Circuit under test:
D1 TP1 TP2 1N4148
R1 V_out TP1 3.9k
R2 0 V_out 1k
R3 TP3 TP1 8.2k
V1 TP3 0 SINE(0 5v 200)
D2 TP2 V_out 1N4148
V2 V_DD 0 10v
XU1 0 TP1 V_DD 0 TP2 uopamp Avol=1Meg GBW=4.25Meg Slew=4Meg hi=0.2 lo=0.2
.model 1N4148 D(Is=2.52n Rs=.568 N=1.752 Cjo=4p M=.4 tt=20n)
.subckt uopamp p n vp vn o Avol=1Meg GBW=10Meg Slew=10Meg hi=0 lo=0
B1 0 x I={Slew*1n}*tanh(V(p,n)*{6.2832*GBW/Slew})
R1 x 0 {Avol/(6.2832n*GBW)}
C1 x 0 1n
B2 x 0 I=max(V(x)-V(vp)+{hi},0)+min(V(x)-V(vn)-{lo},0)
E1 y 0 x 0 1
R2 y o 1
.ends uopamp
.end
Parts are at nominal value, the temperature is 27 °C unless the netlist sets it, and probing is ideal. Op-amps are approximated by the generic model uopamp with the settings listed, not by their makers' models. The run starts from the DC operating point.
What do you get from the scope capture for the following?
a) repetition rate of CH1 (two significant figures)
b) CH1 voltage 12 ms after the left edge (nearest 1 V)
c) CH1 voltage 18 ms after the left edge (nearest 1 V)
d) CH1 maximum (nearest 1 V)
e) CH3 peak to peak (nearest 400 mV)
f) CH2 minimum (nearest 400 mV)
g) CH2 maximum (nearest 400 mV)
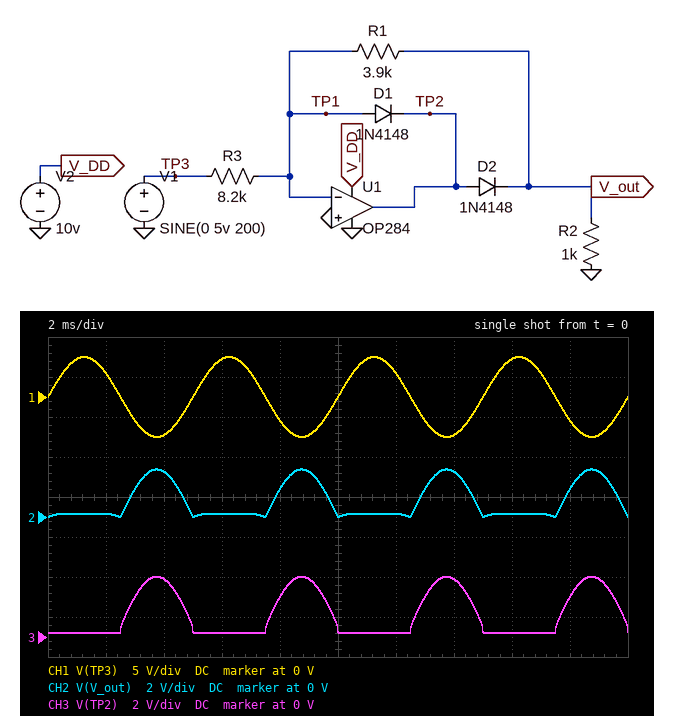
200 Hz
3 V
-3 V
5 V
2.8 V
0 V
2.4 V
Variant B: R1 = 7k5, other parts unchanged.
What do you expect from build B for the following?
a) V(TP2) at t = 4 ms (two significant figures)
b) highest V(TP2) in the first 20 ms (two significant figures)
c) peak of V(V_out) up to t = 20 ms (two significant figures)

5.0 V
5.2 V
4.6 V
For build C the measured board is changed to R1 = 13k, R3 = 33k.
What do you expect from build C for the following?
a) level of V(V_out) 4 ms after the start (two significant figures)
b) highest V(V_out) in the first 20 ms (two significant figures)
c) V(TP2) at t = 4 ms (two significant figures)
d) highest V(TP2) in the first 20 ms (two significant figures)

1.9 V
2.0 V
2.5 V
2.6 V
